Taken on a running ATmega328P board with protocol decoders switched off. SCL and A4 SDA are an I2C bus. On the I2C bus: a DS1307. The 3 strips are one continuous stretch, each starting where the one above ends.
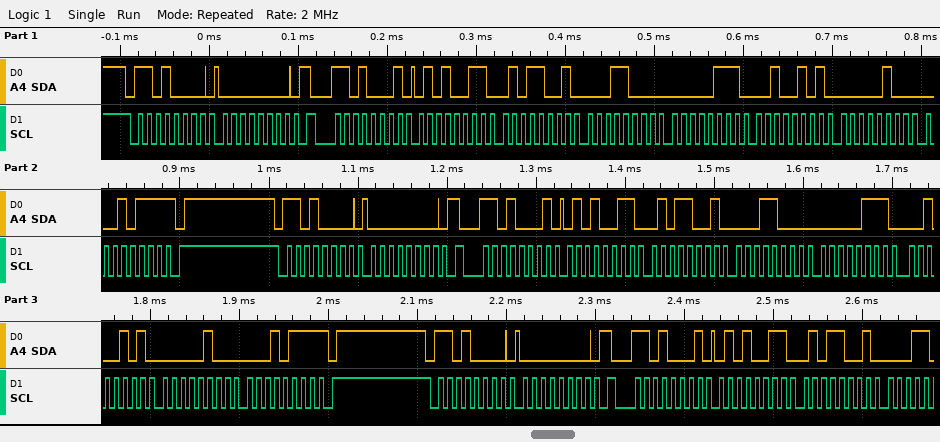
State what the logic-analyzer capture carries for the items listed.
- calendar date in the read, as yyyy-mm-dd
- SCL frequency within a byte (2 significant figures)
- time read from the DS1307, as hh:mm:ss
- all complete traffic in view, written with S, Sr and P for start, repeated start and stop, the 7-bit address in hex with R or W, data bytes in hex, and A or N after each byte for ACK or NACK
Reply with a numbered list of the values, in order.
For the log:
1. 2017-04-25
2. 100 kHz
3. 18:59:53
4. S 68W A 00 A Sr 68R A 53 A 59 A 18 A 07 A 25 A 04 A 17 N P S 68W A 00 A Sr 68R A 53 A 59 A 18 A 07 A 25 A 04 A 17 N P S 68W A 00 A Sr 68R A 53 A 59 A
